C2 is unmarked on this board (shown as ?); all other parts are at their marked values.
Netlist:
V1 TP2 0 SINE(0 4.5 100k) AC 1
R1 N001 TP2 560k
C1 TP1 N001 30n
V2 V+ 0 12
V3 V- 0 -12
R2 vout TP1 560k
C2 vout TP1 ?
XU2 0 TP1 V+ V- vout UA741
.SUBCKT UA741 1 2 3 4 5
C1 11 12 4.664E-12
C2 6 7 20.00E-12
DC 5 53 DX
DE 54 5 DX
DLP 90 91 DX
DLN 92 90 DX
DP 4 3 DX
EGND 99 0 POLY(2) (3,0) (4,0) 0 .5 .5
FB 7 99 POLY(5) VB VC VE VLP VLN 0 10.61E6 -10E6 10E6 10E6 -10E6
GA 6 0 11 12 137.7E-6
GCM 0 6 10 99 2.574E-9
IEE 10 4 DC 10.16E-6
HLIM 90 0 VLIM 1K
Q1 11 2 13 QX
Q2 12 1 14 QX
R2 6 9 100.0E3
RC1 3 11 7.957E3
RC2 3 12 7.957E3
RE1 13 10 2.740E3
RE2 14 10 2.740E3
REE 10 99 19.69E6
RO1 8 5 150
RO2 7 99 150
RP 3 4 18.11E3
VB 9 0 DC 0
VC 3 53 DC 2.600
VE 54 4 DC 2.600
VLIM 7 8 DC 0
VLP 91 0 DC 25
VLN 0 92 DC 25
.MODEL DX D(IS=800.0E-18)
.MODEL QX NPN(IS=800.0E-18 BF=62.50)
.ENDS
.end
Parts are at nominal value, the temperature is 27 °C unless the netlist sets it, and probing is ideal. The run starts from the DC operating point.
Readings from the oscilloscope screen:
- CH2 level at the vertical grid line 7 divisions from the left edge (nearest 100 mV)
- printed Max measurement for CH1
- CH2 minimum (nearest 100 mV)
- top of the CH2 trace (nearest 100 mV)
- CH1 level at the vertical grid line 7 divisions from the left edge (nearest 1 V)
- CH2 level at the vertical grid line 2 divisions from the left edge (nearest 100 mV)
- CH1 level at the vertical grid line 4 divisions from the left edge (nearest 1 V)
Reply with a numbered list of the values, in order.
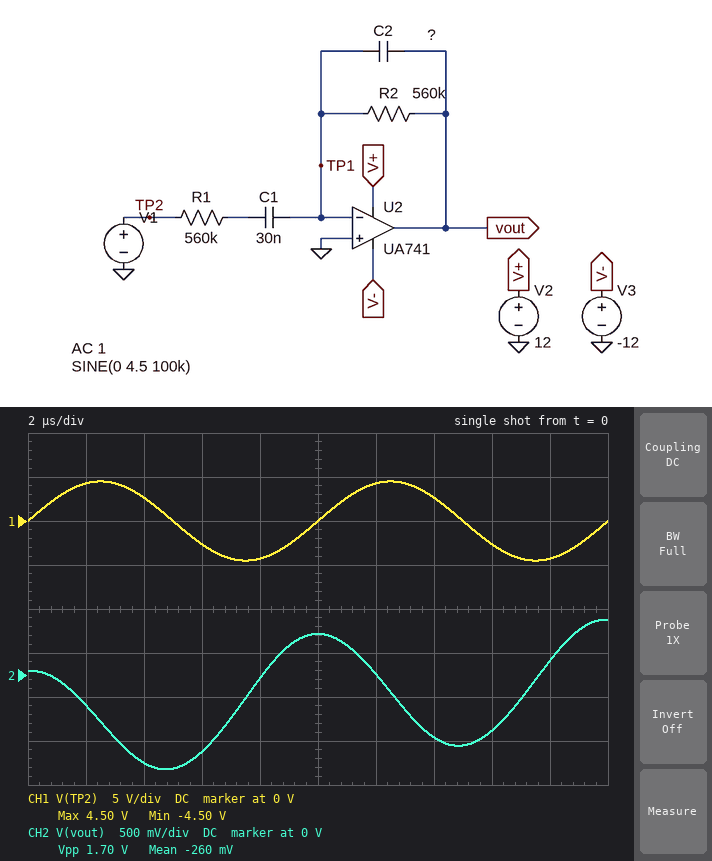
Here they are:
1. -700 mV
2. 4.50 V
3. -1.1 V
4. 600 mV
5. 3 V
6. -1.0 V
7. -4 V
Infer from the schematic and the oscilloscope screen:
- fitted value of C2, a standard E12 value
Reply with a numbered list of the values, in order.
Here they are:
1. 18 pF
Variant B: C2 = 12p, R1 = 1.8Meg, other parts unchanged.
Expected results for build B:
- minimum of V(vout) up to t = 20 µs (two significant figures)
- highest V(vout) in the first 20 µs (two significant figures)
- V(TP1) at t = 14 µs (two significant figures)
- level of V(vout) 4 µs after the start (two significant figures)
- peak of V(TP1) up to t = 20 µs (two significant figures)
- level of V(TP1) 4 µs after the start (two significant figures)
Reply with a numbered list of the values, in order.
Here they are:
1. -430 mV
2. 340 mV
3. 12 mV
4. -410 mV
5. 29 mV
6. 8.8 mV
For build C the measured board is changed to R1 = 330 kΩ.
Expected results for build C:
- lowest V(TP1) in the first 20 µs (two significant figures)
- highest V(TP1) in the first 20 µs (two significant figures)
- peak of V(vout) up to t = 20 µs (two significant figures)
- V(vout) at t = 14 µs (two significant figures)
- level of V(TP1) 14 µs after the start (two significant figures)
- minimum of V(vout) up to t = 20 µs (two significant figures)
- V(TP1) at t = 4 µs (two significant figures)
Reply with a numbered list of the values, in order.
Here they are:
1. -450 mV
2. 270 mV
3. 930 mV
4. -1.1 V
5. 170 mV
6. -1.8 V
7. 80 mV
